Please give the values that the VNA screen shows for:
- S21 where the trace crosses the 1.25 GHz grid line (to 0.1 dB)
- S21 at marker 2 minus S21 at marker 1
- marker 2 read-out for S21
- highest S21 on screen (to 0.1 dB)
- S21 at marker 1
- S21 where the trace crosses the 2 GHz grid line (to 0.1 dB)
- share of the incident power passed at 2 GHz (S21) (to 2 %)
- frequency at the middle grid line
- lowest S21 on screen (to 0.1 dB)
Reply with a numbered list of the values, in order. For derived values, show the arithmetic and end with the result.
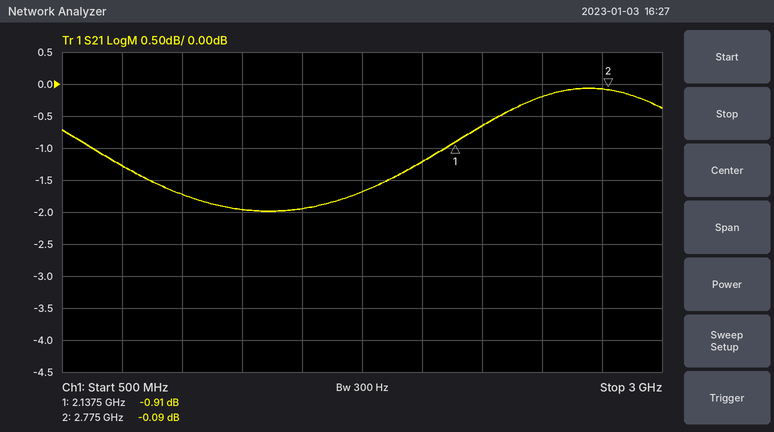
1. -2.0 dB
2. -0.09 − (-0.91) = 0.82 dB
3. -0.09 dB
4. -0.1 dB
5. -0.91 dB
6. -1.2 dB
7. 10^(-1.2/10) ≈ 76 %
8. 1.75 GHz
9. -2.0 dB
